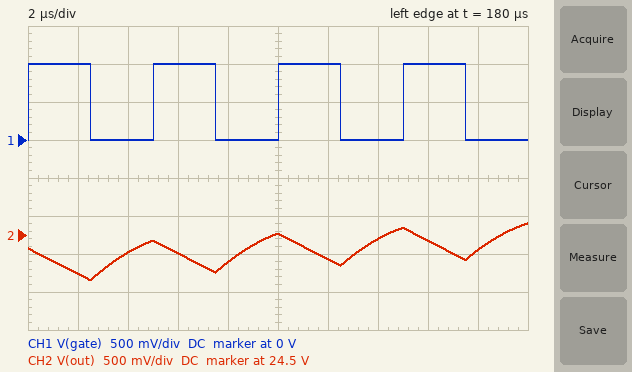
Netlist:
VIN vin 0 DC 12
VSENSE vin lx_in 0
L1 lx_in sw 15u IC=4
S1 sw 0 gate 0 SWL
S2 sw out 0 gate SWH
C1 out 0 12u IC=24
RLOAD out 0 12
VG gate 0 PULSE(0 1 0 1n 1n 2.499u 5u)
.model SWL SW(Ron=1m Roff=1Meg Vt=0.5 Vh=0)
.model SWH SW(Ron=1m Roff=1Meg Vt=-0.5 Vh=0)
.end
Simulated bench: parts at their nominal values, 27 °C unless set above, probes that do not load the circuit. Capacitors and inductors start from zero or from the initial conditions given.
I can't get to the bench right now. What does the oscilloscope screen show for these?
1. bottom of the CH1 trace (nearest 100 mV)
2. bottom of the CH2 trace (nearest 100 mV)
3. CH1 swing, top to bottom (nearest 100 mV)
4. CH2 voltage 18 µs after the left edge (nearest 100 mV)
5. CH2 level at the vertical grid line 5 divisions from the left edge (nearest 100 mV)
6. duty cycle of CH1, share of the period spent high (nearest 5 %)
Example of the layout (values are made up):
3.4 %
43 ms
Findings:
0 V
23.9 V
1.0 V
24.3 V
24.5 V
50 %
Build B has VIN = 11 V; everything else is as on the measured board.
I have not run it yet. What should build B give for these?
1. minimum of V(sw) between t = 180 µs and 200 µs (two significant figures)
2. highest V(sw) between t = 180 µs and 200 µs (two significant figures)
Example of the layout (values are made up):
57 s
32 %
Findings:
2.3 mV
23 V
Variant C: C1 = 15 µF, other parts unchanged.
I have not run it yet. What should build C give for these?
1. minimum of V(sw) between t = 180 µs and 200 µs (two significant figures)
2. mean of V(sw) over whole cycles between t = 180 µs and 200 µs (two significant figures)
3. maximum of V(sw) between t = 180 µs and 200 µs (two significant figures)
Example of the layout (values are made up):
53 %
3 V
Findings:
3.5 mV
12 V
24 V
